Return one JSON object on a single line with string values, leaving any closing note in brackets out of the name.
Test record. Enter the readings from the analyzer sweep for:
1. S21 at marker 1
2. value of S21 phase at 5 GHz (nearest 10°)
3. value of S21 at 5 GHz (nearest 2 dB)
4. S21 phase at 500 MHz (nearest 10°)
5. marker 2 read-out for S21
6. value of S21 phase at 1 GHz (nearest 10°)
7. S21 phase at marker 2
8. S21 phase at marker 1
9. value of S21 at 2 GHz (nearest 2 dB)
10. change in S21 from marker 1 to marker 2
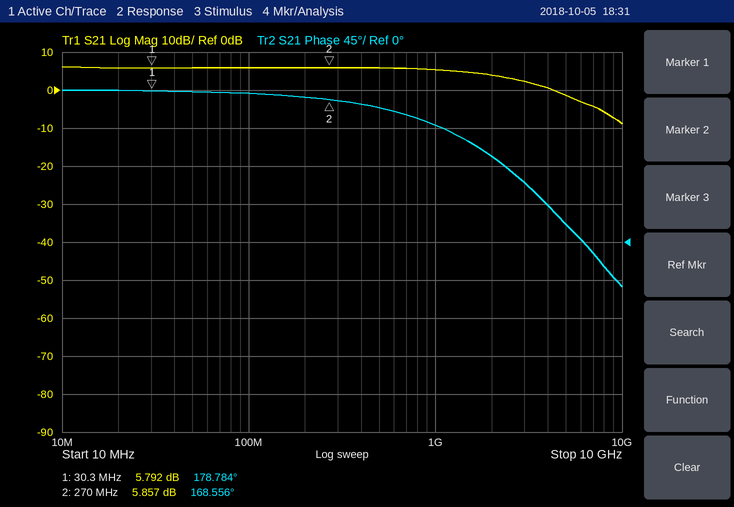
{"S21 at marker 1": "5.792 dB", "value of S21 phase at 5 GHz": "20°", "value of S21 at 5 GHz": "-2 dB", "S21 phase at 500 MHz": "160°", "marker 2 read-out for S21": "5.857 dB", "value of S21 phase at 1 GHz": "140°", "S21 phase at marker 2": "168.556°", "S21 phase at marker 1": "178.784°", "value of S21 at 2 GHz": "4 dB", "change in S21 from marker 1 to marker 2": "0.065 dB"}
